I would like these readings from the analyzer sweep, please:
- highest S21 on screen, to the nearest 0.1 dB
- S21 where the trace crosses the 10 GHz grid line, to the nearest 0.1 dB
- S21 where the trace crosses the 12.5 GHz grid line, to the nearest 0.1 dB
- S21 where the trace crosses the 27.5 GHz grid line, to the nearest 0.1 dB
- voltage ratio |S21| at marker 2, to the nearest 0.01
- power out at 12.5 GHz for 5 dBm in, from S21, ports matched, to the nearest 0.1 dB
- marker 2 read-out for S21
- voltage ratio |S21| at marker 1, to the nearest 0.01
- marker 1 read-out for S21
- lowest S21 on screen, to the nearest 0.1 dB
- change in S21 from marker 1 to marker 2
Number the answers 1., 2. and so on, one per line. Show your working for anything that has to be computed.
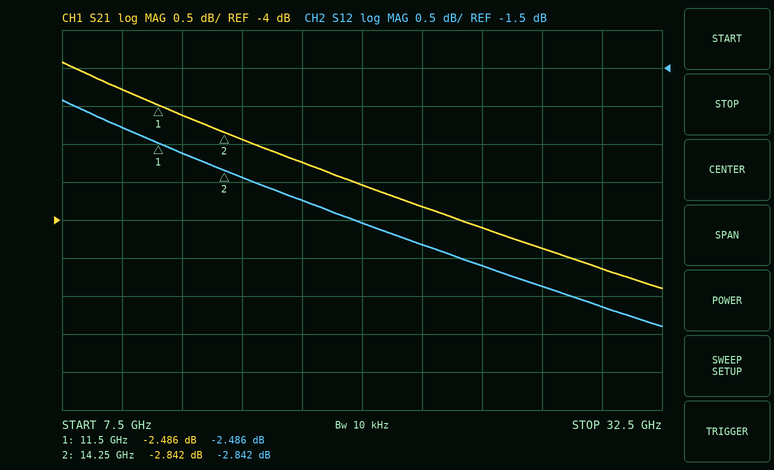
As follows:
1. -1.9 dB
2. -2.3 dB
3. -2.6 dB
4. -4.4 dB
5. 10^(-2.842/20) ≈ 0.72
6. 5 dBm + (-2.6 dB) = 2.4 dBm
7. -2.842 dB
8. 10^(-2.486/20) ≈ 0.75
9. -2.486 dB
10. -4.9 dB
11. -2.842 − (-2.486) = -0.356 dB
